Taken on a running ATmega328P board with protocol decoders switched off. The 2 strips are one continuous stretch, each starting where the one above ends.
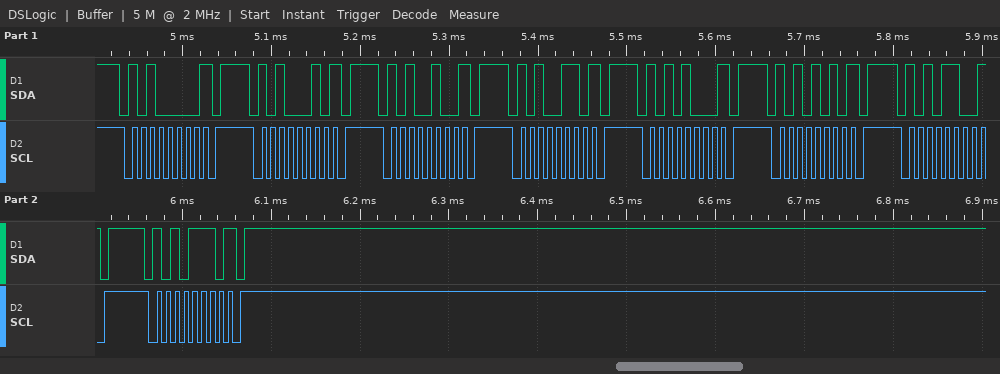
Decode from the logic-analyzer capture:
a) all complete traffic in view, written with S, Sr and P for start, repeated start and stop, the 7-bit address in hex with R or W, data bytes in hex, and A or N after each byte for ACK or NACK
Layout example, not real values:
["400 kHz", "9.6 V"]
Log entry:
["S 50W N P S 51W N P S 52W N P S 53W N P S 54W N P S 55W N P S 56W N P S 57W N P"]
